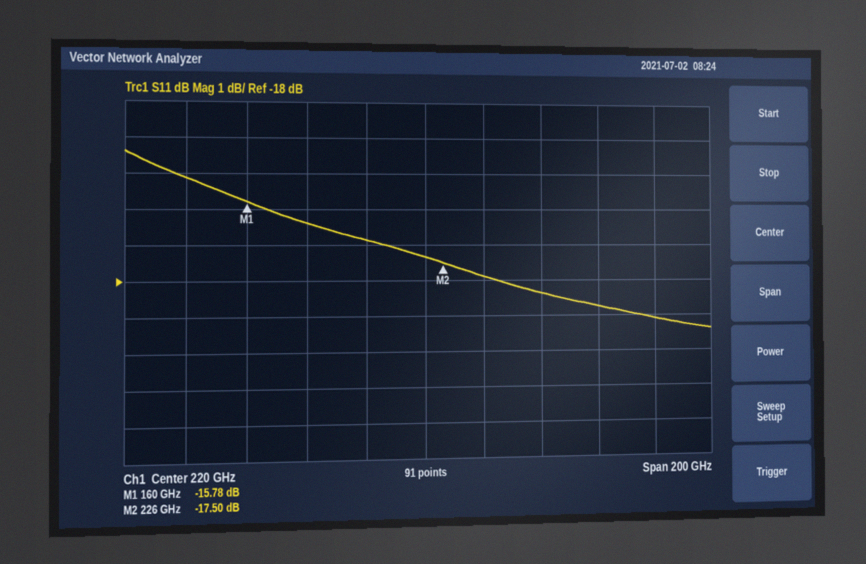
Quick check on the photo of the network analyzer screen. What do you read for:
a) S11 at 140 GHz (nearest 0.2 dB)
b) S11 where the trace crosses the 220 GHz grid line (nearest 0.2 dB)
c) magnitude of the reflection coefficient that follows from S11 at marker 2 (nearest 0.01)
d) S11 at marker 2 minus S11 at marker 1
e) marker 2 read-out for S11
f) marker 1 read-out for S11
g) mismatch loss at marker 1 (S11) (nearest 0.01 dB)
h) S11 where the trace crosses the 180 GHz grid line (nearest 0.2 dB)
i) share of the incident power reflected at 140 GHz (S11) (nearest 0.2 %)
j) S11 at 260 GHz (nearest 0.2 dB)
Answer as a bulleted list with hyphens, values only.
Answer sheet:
- -15.2 dB
- -17.4 dB
- 0.13
- -1.72 dB
- -17.50 dB
- -15.78 dB
- 0.12 dB
- -16.4 dB
- 3.0 %
- -18.4 dB
